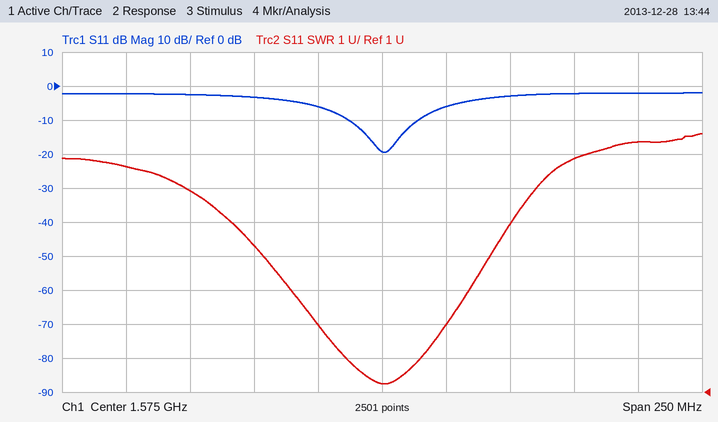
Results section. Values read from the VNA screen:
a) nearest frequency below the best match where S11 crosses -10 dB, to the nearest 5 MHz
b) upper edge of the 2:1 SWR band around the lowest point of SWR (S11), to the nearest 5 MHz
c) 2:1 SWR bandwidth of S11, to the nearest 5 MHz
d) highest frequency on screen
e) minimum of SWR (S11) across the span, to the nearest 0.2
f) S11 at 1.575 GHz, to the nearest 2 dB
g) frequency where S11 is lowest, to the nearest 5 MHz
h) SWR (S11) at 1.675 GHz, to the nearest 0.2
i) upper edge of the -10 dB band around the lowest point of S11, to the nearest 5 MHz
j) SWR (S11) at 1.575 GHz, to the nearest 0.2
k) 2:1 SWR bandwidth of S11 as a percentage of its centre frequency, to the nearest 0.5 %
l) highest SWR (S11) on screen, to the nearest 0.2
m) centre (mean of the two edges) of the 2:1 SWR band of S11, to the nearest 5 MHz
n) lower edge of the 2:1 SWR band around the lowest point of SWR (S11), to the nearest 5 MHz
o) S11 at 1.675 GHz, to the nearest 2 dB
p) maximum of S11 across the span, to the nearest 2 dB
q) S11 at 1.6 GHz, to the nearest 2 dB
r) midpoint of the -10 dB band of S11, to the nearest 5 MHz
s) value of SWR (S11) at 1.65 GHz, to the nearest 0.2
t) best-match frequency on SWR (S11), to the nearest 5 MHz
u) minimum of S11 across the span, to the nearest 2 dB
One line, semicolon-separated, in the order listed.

1.560 GHz; 1.590 GHz; 30 MHz; 1.7 GHz; 1.2; -20 dB; 1.575 GHz; 8.4; 1.590 GHz; 1.2; 2.0 %; 8.6; 1.575 GHz; 1.560 GHz; -2 dB; -2 dB; -6 dB; 1.575 GHz; 7.8; 1.575 GHz; -20 dB
